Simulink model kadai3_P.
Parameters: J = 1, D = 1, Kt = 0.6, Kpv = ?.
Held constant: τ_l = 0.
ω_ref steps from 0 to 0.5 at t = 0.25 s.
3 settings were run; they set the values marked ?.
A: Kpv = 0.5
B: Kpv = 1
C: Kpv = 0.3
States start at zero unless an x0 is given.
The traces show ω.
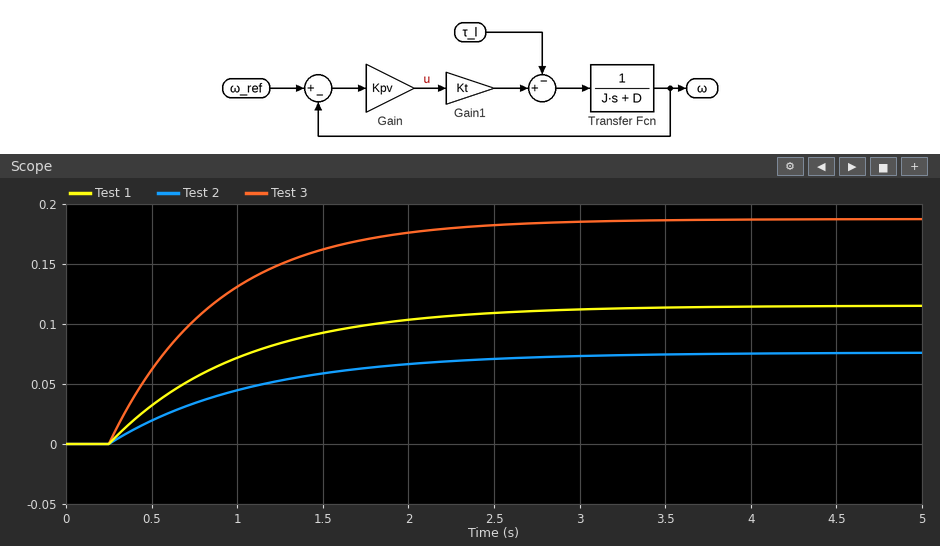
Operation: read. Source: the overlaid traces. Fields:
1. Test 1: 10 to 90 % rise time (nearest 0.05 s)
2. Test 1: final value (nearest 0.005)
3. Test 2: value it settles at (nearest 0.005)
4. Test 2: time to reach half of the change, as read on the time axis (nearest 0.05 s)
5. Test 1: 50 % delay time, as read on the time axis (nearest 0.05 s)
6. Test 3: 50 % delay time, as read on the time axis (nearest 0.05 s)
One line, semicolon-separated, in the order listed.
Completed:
1.70 s; 0.115; 0.075; 0.85 s; 0.80 s; 0.70 s
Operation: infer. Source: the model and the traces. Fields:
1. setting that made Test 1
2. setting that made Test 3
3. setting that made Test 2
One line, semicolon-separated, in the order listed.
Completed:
A; B; C
